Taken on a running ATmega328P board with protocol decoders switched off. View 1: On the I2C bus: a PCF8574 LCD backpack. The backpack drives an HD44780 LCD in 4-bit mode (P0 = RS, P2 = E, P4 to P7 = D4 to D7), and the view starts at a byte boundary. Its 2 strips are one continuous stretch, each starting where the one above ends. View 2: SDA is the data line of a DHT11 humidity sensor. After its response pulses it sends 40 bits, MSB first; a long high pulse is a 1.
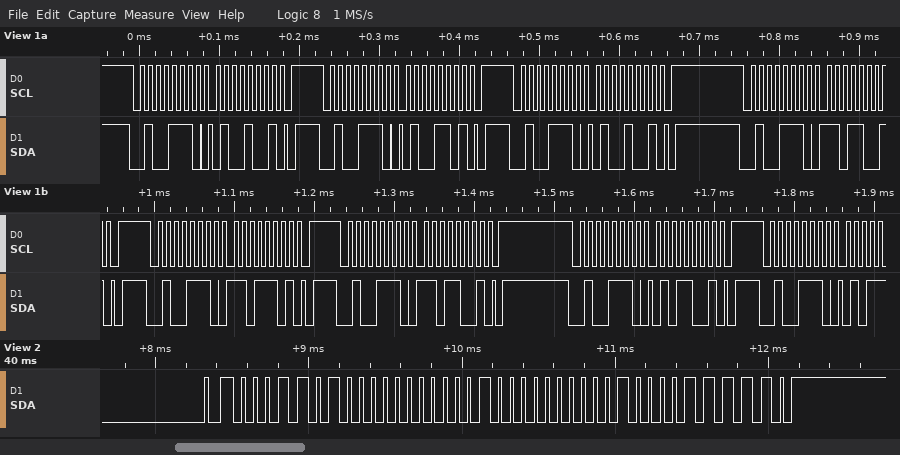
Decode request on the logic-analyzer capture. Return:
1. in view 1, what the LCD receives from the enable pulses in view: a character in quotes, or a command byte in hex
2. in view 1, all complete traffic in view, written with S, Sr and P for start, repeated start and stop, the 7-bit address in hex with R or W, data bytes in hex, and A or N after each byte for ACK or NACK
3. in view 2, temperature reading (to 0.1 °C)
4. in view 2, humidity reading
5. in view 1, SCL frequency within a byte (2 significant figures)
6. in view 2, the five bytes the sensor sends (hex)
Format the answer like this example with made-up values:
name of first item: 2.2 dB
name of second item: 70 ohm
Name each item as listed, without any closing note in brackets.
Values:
in view 1, what the LCD receives from the enable pulses in view: a character in quotes, or a command byte in hex: 'M'
in view 1, all complete traffic in view, written with S, Sr and P for start, repeated start and stop, the 7-bit address in hex with R or W, data bytes in hex, and A or N after each byte for ACK or NACK: S 27W A 49 A P S 27W A 4D A P S 27W A 49 A P S 27W A D9 A P S 27W A DD A P S 27W A D9 A P S 27W A 59 A P S 27W A
in view 2, temperature reading: 32.4 °C
in view 2, humidity reading: 26 %
in view 1, SCL frequency within a byte: 100 kHz
in view 2, the five bytes the sensor sends: 1A 00 20 04 3E
